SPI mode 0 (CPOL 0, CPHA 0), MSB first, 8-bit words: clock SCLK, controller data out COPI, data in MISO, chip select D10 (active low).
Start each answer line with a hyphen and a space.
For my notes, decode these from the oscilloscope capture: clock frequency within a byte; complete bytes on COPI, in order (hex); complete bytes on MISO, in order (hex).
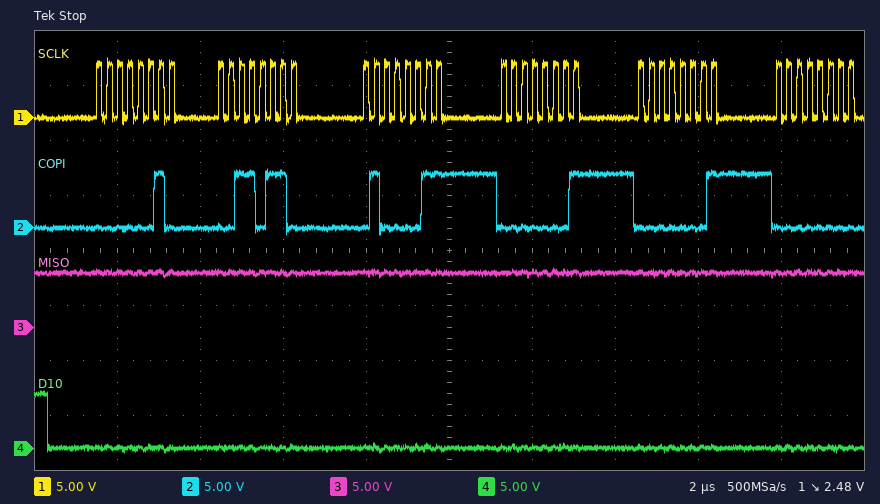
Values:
- 4 MHz
- 02 36 43 01 01 00
- FF FF FF FF FF FF
